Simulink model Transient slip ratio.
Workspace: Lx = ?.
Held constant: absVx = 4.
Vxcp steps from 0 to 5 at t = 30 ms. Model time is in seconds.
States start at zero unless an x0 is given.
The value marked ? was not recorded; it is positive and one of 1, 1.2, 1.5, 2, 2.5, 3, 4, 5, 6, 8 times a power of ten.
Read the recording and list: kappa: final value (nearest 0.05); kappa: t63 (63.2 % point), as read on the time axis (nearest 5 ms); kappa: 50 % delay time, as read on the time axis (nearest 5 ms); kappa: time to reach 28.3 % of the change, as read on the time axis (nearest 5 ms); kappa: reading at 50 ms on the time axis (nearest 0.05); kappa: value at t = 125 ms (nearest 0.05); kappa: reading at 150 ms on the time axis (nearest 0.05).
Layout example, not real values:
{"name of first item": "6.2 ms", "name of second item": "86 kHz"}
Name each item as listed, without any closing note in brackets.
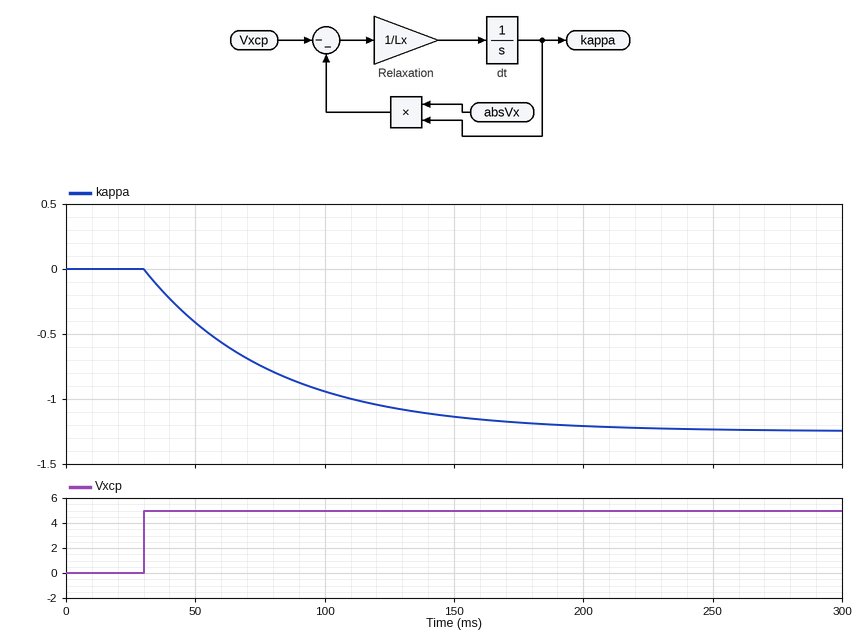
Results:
{"kappa: final value": "-1.25", "kappa: t63 (63.2 % point), as read on the time axis": "80 ms", "kappa: 50 % delay time, as read on the time axis": "65 ms", "kappa: time to reach 28.3 % of the change, as read on the time axis": "45 ms", "kappa: reading at 50 ms on the time axis": "-0.40", "kappa: value at t = 125 ms": "-1.05", "kappa: reading at 150 ms on the time axis": "-1.15"}
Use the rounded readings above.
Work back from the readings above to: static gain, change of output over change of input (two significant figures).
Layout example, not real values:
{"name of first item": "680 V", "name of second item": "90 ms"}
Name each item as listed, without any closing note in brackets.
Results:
{"static gain, change of output over change of input": "-0.25"}
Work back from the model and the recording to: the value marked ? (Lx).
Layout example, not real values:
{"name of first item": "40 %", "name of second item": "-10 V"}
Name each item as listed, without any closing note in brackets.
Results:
{"the value marked ?": "0.2"}
